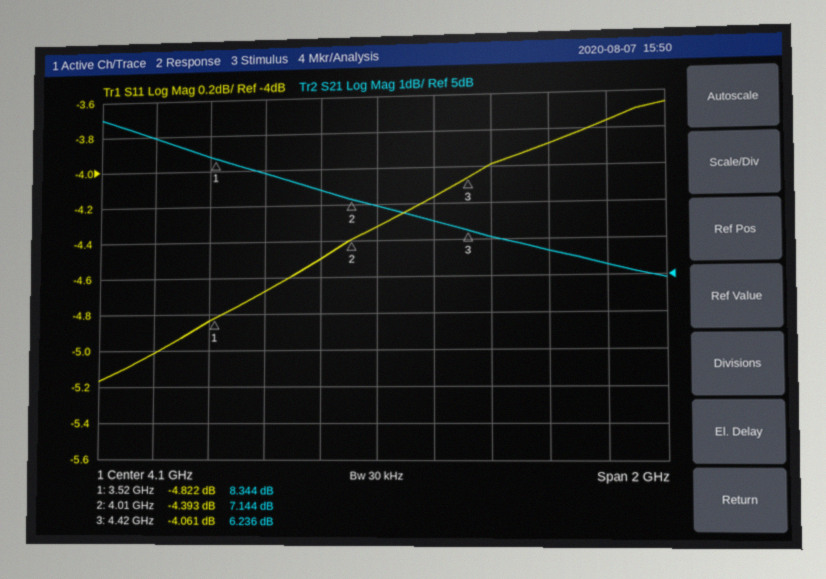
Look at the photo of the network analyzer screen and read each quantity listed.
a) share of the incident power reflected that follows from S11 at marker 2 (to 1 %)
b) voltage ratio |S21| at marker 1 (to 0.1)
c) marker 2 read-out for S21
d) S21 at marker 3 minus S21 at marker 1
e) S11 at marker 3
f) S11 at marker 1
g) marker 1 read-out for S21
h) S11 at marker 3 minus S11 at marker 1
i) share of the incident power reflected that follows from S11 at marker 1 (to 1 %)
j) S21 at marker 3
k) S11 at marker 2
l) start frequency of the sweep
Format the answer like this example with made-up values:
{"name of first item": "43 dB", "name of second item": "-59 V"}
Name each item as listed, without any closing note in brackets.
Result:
{"share of the incident power reflected that follows from S11 at marker 2": "36 %", "voltage ratio |S21| at marker 1": "2.6", "marker 2 read-out for S21": "7.144 dB", "S21 at marker 3 minus S21 at marker 1": "-2.108 dB", "S11 at marker 3": "-4.061 dB", "S11 at marker 1": "-4.822 dB", "marker 1 read-out for S21": "8.344 dB", "S11 at marker 3 minus S11 at marker 1": "0.761 dB", "share of the incident power reflected that follows from S11 at marker 1": "33 %", "S21 at marker 3": "6.236 dB", "S11 at marker 2": "-4.393 dB", "start frequency of the sweep": "3.1 GHz"}
